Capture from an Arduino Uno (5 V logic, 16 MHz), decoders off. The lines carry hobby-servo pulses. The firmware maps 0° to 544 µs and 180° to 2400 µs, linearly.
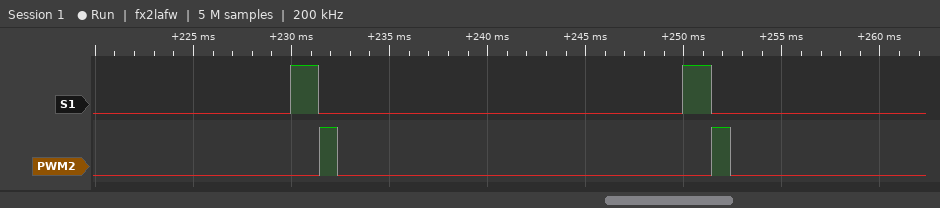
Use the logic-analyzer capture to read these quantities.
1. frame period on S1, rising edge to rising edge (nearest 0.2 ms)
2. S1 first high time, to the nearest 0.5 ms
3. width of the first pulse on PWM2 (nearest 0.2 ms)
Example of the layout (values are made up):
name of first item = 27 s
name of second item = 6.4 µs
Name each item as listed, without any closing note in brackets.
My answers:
frame period on S1, rising edge to rising edge = 20.0 ms
S1 first high time, to the nearest 0.5 ms = 1.5 ms
width of the first pulse on PWM2 = 1.0 ms
